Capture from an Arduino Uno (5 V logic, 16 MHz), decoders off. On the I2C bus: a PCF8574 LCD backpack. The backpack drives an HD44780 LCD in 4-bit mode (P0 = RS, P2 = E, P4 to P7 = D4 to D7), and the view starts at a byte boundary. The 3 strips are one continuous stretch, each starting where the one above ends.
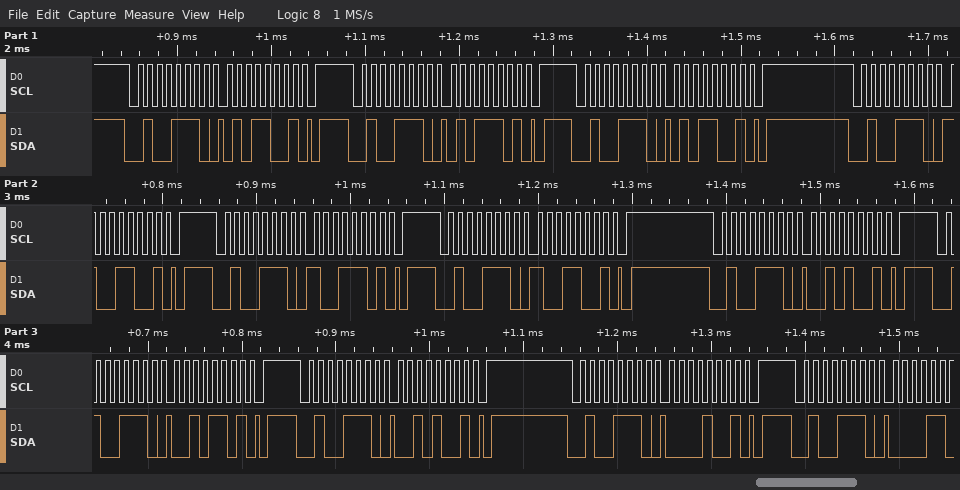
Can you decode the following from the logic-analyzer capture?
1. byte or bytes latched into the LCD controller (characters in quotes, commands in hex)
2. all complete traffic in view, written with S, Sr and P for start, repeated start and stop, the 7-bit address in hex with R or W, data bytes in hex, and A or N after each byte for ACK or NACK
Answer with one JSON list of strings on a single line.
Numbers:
["'Y'", "S 27W A 59 A P S 27W A 5D A P S 27W A 59 A P S 27W A 99 A P S 27W A 9D A P S 27W A 99 A P S 27W A 29 A P S 27W A 2D A P S 27W A 29 A P S 27W A 09 A P S 27W A"]
